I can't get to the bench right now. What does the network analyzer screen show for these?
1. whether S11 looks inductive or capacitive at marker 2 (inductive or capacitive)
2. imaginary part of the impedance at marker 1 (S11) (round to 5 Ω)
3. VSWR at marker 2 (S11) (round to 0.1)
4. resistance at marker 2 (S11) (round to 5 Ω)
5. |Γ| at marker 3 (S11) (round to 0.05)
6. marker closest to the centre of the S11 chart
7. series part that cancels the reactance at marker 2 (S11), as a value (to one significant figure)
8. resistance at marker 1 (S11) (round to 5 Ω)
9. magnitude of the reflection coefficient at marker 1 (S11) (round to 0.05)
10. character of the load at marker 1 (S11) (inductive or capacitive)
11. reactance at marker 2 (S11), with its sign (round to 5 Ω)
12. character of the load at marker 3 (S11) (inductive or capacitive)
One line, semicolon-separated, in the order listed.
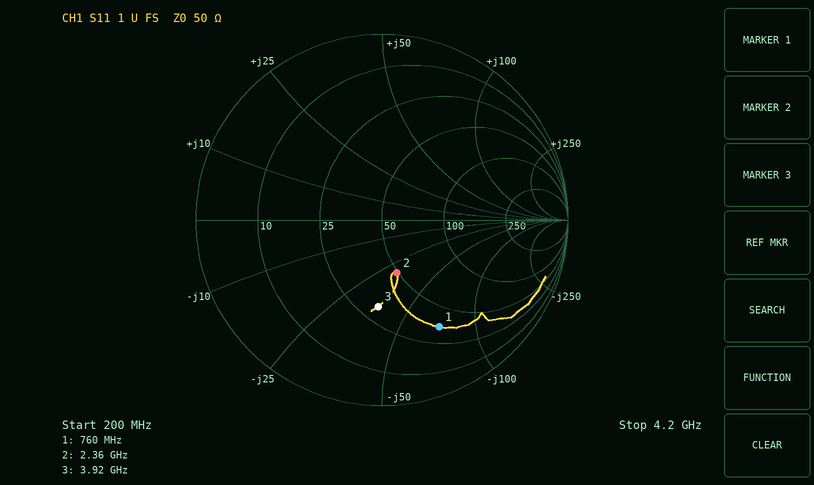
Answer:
capacitive; -70 Ω; 1.8; 50 Ω; 0.45; marker 2; 2 nH; 35 Ω; 0.65; capacitive; -30 Ω; capacitive
